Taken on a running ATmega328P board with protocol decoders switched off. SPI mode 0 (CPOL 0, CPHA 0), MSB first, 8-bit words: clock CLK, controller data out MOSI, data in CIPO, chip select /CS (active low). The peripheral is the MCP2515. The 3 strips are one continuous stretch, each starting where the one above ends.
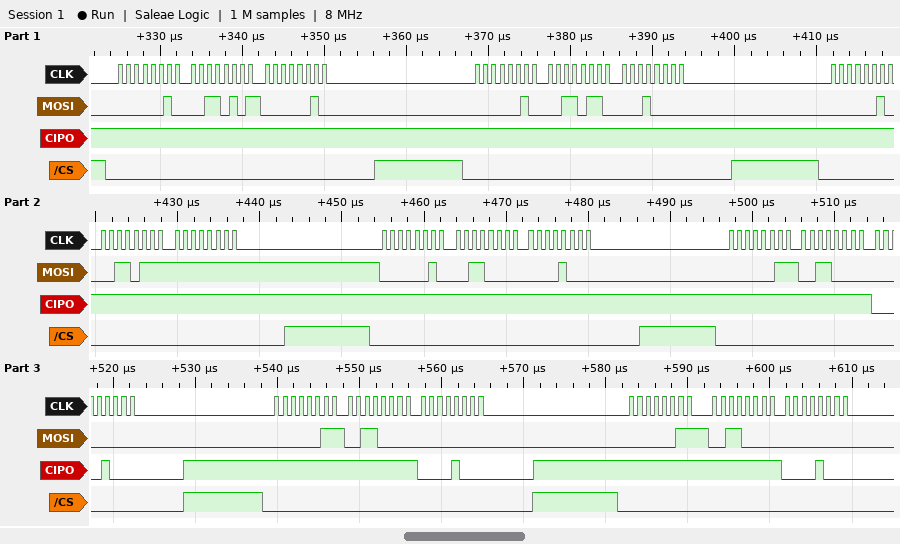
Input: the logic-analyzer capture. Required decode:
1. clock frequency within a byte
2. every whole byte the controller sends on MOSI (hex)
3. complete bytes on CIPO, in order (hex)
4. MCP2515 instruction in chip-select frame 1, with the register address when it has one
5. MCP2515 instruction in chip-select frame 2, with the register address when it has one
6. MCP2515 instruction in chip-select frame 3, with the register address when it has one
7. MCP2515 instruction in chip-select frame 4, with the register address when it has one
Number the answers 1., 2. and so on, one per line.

1. 1 MHz
2. 0x02 0x35 0x02 0x02 0x36 0x10 0x02 0x37 0xFF 0x02 0x30 0x08 0x03 0x30 0x00 0x03 0x30 0x00 0x03 0x30 0x00
3. 0xFF 0xFF 0xFF 0xFF 0xFF 0xFF 0xFF 0xFF 0xFF 0xFF 0xFF 0xFF 0xFF 0xFF 0x08 0xFF 0xFF 0x08 0xFF 0xFF 0x08
4. WRITE 0x35
5. WRITE 0x36
6. WRITE 0x37
7. WRITE 0x30
